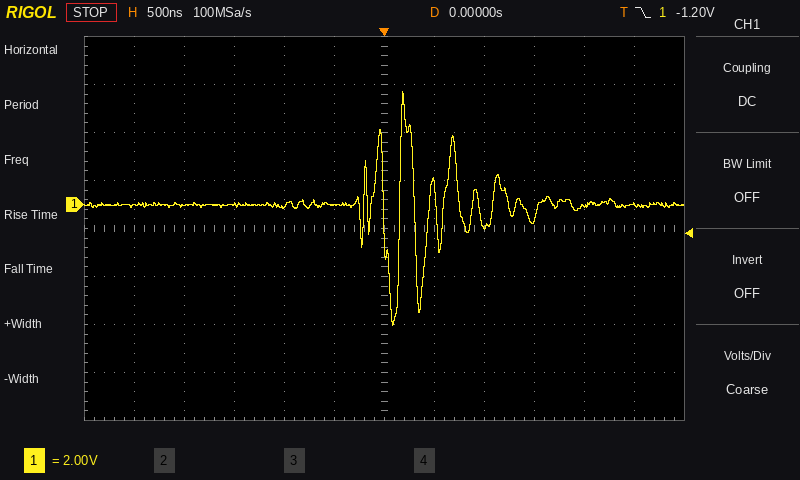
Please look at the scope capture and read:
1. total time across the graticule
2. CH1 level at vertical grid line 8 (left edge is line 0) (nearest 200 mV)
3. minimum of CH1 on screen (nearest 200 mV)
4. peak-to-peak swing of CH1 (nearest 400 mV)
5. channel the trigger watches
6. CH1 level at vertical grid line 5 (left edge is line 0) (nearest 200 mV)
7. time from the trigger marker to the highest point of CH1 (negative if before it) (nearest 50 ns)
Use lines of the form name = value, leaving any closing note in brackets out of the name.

total time across the graticule = 6 µs
CH1 level at vertical grid line 8 (left edge is line 0) = -800 mV
minimum of CH1 on screen = -5.0 V
peak-to-peak swing of CH1 = 9.6 V
channel the trigger watches = CH1
CH1 level at vertical grid line 5 (left edge is line 0) = 0.0 V
time from the trigger marker to the highest point of CH1 (negative if before it) = +200 ns
